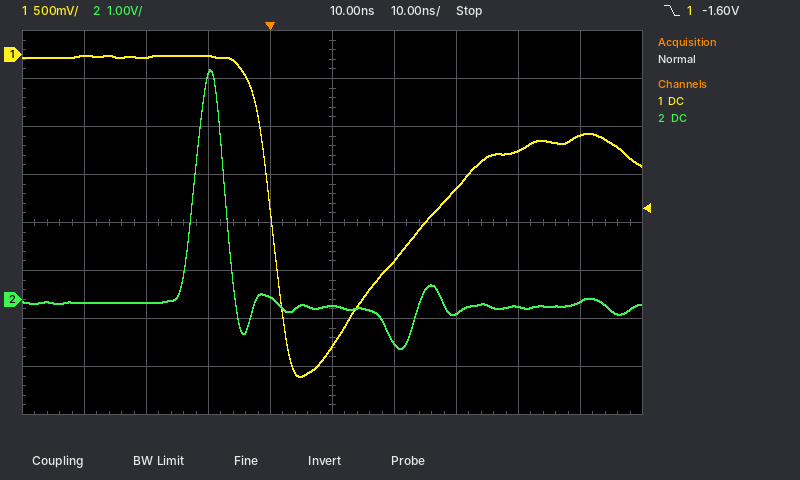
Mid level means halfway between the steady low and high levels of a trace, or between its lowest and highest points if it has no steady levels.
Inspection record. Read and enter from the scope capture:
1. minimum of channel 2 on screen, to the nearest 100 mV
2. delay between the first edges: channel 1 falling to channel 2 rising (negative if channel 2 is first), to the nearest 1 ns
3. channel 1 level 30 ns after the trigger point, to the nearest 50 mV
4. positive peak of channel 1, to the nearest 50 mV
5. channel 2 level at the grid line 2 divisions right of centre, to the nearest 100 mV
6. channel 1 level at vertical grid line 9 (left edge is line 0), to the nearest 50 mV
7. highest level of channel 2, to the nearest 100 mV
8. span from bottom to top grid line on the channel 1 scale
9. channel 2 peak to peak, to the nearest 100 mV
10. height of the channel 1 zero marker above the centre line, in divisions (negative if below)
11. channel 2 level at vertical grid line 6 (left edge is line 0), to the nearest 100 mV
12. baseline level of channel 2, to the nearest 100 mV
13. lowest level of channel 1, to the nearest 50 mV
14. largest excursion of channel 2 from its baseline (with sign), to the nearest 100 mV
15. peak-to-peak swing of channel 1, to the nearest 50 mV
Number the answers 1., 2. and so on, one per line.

1. -1.0 V
2. -13 ns
3. -1.40 V
4. 0 mV
5. -300 mV
6. -850 mV
7. 4.8 V
8. 4 V
9. 5.8 V
10. +3.5 div
11. -900 mV
12. -100 mV
13. -3.35 V
14. +4.9 V
15. 3.35 V
